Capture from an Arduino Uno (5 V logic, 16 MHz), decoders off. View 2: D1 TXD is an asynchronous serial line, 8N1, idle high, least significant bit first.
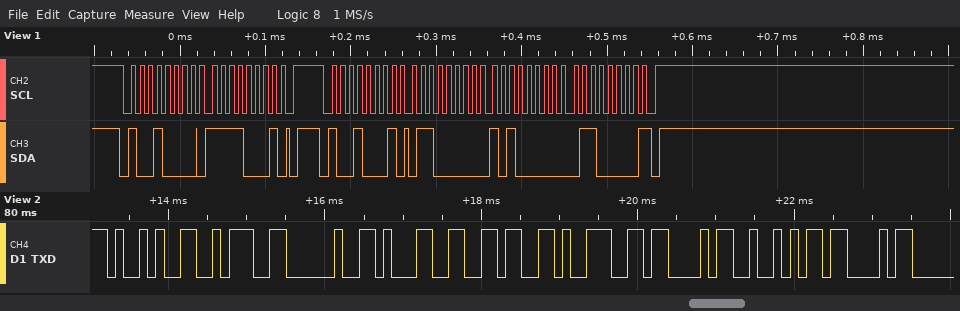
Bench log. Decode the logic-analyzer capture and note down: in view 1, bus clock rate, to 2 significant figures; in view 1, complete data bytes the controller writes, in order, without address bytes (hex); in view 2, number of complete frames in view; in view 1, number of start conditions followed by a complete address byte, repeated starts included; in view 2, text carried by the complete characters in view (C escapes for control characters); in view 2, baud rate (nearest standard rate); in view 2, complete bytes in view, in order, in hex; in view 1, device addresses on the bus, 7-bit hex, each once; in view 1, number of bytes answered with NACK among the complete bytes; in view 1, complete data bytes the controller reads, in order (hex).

100 kHz
F1
9
2
"): 169CRC"
9600 baud
29 3A 20 31 36 39 43 52 43
0x48
1
60 A0 60
